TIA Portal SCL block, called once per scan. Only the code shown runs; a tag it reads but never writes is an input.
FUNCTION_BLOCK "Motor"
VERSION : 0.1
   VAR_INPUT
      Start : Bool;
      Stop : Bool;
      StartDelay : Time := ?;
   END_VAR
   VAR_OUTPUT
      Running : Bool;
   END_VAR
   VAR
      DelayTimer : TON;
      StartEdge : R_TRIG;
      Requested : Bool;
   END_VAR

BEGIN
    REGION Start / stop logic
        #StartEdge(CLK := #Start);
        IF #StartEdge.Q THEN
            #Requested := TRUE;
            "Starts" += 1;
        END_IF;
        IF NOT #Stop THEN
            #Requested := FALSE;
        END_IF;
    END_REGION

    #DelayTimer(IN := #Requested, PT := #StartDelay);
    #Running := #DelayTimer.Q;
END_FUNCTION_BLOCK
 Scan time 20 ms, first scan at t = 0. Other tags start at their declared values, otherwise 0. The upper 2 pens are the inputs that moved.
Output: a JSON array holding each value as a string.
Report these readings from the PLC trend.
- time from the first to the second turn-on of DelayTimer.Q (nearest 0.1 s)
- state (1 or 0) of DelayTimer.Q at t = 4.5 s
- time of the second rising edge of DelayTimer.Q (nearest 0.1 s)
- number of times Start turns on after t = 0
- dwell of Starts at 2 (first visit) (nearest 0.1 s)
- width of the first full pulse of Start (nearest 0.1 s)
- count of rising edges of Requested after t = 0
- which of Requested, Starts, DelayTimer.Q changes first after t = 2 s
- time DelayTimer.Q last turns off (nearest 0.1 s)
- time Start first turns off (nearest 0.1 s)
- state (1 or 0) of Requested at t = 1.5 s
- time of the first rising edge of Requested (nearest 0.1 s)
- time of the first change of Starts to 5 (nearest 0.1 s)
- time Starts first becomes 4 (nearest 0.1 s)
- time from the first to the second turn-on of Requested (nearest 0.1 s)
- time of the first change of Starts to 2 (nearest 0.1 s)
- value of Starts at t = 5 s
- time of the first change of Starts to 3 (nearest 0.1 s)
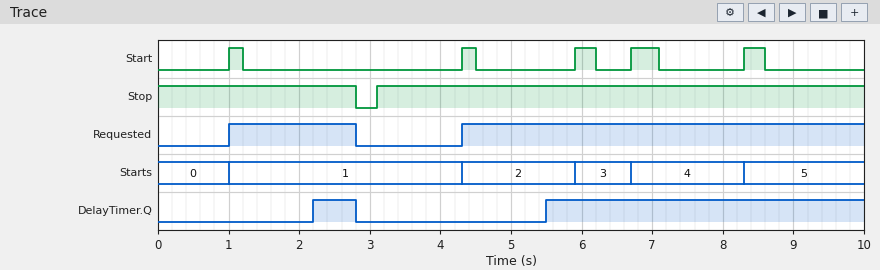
["3.3 s", "0", "5.5 s", "5", "1.6 s", "0.2 s", "2", "DelayTimer.Q", "2.8 s", "1.2 s", "1", "1.0 s", "8.3 s", "6.7 s", "3.3 s", "4.3 s", "2", "5.9 s"]
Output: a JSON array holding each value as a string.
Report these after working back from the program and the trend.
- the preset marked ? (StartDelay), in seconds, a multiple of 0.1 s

["1.2 s"]
